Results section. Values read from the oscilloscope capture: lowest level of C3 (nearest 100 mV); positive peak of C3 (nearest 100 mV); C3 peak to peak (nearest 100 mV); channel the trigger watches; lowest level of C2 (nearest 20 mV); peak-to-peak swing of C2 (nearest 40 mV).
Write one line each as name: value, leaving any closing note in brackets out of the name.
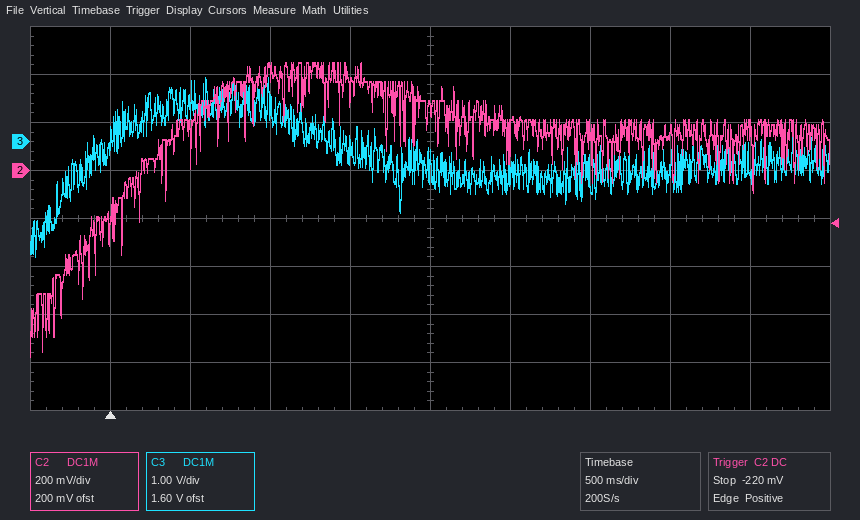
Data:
lowest level of C3: -2.4 V
positive peak of C3: 1.3 V
C3 peak to peak: 3.7 V
channel the trigger watches: C2
lowest level of C2: -780 mV
peak-to-peak swing of C2: 1.24 V
